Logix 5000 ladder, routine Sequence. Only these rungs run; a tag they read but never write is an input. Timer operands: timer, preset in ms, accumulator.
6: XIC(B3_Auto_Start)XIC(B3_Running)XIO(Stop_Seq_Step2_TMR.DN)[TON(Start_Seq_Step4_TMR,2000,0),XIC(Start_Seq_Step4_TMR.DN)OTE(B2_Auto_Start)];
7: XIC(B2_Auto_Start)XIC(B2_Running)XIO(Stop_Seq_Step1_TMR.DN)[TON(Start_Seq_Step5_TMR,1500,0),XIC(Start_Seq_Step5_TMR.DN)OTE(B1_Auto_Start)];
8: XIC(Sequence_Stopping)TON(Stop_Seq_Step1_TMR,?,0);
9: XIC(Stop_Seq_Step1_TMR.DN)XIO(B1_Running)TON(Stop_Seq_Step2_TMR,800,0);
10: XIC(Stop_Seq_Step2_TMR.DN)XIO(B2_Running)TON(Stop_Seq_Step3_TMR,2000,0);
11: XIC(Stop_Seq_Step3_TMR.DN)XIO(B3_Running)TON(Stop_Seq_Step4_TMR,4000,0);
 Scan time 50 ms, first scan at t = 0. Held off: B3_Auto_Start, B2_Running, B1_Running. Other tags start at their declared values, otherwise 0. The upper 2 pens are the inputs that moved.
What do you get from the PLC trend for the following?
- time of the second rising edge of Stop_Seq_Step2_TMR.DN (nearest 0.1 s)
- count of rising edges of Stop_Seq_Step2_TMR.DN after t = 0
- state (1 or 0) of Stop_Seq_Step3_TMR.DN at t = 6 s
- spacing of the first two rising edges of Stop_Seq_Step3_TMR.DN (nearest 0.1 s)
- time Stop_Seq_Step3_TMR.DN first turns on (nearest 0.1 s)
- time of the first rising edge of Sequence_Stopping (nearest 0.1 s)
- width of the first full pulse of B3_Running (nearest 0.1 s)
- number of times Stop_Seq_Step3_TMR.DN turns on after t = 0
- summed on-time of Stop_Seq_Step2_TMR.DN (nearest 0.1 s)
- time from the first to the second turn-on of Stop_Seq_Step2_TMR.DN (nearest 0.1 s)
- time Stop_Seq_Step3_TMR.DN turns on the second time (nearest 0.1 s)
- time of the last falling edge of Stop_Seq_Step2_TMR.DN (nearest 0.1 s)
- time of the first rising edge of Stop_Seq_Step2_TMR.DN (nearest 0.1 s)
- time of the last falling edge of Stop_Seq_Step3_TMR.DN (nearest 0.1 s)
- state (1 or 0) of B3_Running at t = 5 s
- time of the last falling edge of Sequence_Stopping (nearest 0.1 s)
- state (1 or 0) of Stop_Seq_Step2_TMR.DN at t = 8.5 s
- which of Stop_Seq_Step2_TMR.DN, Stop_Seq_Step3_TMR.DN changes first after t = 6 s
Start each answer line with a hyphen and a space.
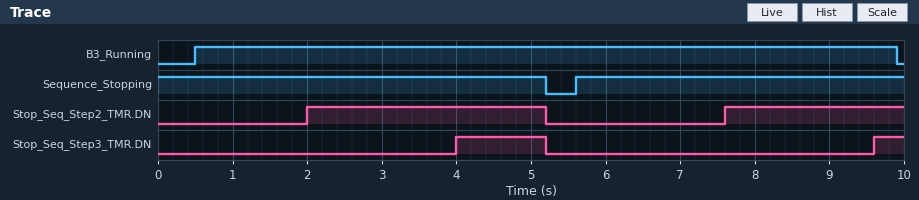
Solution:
- 7.6 s
- 2
- 0
- 5.6 s
- 4.0 s
- 5.6 s
- 9.4 s
- 2
- 5.6 s
- 5.6 s
- 9.6 s
- 5.2 s
- 2.0 s
- 5.2 s
- 1
- 5.2 s
- 1
- Stop_Seq_Step2_TMR.DN
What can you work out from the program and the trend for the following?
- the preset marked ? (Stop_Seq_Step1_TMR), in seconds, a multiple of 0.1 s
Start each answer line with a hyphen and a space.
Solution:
- 1.2 s
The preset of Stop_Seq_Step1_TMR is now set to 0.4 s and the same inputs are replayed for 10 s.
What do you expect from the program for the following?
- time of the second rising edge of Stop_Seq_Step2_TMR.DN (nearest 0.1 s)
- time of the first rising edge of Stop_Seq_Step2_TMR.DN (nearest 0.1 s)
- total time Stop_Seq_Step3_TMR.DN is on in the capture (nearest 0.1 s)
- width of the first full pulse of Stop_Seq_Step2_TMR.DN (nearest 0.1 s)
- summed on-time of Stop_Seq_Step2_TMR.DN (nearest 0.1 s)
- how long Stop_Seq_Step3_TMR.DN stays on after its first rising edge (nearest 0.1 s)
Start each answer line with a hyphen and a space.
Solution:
- 6.8 s
- 1.2 s
- 3.2 s
- 4.0 s
- 7.2 s
- 2.0 s
